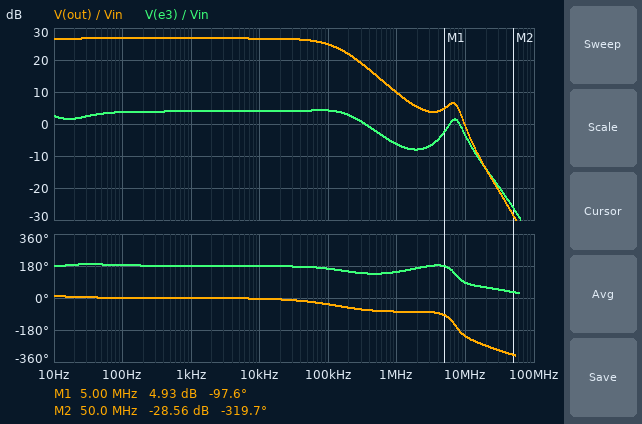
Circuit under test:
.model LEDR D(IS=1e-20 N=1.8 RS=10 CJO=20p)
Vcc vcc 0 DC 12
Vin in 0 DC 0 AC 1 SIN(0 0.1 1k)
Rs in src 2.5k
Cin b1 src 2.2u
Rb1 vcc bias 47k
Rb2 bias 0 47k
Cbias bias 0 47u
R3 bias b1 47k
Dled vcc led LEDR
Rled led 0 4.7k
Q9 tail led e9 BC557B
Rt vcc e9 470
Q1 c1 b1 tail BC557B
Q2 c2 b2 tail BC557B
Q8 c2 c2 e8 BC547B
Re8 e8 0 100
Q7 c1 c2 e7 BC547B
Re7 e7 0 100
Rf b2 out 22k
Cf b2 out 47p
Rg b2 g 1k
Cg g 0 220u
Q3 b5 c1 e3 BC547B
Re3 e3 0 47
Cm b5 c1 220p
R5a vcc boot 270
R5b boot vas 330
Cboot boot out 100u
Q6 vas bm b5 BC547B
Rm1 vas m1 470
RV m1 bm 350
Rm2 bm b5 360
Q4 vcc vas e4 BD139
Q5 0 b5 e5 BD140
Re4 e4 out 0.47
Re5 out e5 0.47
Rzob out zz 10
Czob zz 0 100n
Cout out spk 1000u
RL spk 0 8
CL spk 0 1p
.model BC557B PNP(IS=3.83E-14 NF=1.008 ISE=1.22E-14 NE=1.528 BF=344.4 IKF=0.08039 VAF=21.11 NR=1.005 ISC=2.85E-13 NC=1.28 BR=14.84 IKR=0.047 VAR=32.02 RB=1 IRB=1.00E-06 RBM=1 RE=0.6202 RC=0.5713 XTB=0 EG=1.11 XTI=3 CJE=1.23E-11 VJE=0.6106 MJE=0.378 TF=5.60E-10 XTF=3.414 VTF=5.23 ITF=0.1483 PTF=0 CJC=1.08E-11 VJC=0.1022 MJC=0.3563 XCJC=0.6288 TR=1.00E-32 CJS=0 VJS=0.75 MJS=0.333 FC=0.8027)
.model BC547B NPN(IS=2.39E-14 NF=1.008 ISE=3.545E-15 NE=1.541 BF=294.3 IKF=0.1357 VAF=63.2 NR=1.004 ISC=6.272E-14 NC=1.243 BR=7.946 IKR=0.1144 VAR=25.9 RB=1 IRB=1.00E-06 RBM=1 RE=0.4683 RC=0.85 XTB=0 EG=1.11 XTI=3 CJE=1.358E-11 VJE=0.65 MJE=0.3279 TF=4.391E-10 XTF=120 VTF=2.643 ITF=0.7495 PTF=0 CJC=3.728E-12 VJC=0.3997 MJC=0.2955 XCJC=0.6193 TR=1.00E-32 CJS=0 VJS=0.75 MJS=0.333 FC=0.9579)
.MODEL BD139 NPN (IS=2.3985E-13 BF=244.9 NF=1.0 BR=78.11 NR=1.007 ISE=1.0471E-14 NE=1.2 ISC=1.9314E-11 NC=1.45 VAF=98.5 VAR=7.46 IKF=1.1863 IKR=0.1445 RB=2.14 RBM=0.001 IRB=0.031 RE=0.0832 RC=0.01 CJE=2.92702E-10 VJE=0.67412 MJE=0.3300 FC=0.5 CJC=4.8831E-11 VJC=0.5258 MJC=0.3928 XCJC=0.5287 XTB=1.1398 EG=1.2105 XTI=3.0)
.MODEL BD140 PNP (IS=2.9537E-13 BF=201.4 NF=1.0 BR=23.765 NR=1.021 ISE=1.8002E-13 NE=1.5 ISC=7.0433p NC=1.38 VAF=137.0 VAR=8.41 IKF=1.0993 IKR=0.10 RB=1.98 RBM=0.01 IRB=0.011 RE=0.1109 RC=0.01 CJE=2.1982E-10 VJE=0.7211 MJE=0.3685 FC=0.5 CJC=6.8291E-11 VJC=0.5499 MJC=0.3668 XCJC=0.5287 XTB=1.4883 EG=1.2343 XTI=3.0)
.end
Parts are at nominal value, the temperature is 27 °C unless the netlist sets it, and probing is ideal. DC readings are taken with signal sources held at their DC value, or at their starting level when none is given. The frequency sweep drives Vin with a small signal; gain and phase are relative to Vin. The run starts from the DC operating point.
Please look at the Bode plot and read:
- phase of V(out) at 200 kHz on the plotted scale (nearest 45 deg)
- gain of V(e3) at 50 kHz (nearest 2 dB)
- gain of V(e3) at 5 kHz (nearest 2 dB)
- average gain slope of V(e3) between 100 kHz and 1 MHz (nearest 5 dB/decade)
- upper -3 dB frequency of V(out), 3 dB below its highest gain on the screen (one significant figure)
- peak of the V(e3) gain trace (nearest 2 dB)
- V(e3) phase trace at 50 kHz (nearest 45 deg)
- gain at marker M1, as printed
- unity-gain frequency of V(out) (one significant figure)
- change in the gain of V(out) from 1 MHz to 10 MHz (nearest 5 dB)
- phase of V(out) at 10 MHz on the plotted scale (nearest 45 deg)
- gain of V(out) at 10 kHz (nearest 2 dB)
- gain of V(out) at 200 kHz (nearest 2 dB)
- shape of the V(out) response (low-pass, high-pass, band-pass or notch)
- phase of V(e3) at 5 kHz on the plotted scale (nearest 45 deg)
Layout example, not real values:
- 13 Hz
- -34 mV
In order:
- -45 deg
- 4 dB
- 4 dB
- -10 dB/decade
- 100 kHz
- 4 dB
- 180 deg
- 4.93 dB
- 10 MHz
- -10 dB
- -225 deg
- 26 dB
- 22 dB
- low-pass
- 180 deg
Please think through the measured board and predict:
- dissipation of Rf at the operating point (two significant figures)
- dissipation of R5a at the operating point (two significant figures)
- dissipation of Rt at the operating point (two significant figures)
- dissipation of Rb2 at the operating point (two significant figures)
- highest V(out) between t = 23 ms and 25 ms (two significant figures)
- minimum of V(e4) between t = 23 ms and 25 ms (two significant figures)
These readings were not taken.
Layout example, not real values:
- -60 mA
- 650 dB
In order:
- 220 nW
- 17 mW
- 3.2 mW
- 790 µW
- 8.3 V
- 4.2 V
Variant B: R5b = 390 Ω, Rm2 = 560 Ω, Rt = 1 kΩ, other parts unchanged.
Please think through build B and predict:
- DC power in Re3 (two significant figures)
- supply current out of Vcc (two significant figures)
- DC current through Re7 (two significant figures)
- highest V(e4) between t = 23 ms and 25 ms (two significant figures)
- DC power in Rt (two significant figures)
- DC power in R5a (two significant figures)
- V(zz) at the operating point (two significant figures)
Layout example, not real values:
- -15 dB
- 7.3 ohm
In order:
- 2.9 mW
- 240 mA
- 610 µA
- 8.4 V
- 1.6 mW
- 16 mW
- 6.1 V
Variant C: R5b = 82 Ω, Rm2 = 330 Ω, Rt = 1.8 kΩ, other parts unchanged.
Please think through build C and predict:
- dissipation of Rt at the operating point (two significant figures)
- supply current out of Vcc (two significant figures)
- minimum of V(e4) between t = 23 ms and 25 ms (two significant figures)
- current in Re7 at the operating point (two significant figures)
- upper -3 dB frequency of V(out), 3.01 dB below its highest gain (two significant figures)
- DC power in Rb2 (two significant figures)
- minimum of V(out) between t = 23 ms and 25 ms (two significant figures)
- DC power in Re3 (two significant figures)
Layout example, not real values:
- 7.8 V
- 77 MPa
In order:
- 890 µW
- 780 mA
- 4.2 V
- 320 µA
- 110 kHz
- 770 µW
- 3.9 V
- 10 mW
